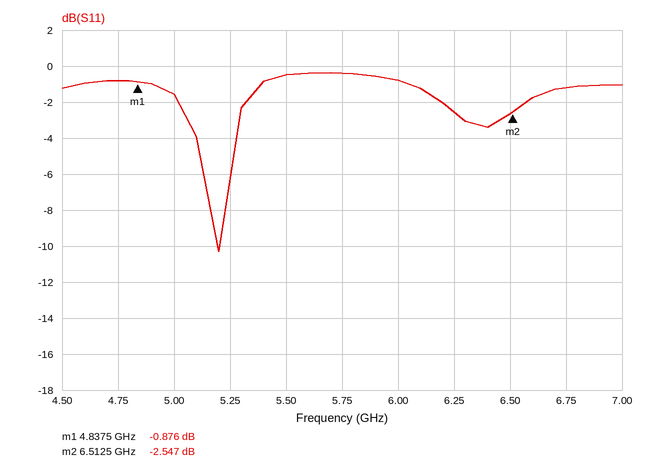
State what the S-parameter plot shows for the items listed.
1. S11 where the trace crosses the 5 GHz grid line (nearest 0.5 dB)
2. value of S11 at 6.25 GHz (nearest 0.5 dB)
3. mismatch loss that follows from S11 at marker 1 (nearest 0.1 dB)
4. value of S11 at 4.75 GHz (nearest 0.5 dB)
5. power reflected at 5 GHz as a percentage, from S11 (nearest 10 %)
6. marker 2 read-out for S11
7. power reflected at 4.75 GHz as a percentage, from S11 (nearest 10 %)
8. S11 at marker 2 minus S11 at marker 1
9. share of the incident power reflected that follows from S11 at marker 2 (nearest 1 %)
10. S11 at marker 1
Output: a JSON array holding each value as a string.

["-1.5 dB", "-2.5 dB", "7.4 dB", "-1.0 dB", "70 %", "-2.547 dB", "80 %", "-1.671 dB", "56 %", "-0.876 dB"]
